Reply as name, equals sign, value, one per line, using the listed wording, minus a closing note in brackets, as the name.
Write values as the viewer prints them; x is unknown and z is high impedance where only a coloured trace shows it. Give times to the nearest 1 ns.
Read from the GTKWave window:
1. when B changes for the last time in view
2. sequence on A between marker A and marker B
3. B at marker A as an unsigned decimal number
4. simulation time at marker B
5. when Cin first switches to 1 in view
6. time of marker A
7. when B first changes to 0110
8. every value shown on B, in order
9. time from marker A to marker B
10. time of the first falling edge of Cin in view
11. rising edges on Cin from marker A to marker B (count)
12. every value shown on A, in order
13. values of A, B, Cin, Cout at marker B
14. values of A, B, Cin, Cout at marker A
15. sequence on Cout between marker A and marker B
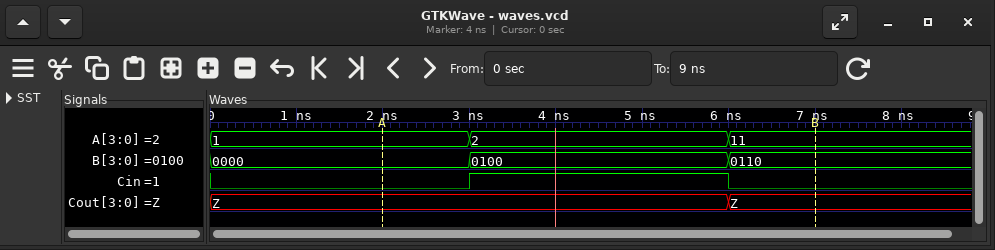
when B changes for the last time in view = 6 ns
sequence on A between marker A and marker B = 1, 2, 11
B at marker A as an unsigned decimal number = 0
simulation time at marker B = 7 ns
when Cin first switches to 1 in view = 3 ns
time of marker A = 2 ns
when B first changes to 0110 = 6 ns
every value shown on B, in order = 0000, 0100, 0110
time from marker A to marker B = 5 ns
time of the first falling edge of Cin in view = 6 ns
rising edges on Cin from marker A to marker B = 1
every value shown on A, in order = 1, 2, 11
values of A, B, Cin, Cout at marker B = A=11, B=0110, Cin=0, Cout=Z
values of A, B, Cin, Cout at marker A = A=1, B=0000, Cin=0, Cout=Z
sequence on Cout between marker A and marker B = Z, Z
